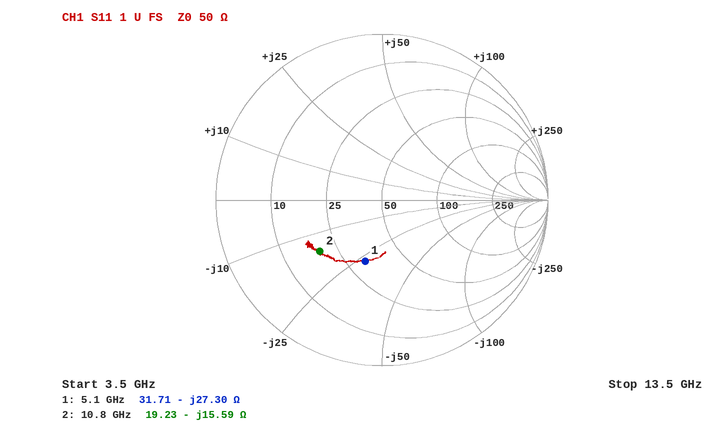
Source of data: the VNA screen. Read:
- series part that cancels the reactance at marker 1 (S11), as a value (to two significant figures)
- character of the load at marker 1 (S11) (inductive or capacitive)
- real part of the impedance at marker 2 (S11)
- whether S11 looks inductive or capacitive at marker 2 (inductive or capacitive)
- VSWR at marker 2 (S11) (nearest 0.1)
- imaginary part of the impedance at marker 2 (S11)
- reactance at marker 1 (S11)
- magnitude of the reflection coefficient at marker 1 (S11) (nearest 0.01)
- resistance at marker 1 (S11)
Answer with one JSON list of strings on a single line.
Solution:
["850 pH", "capacitive", "19.23 Ω", "capacitive", "2.9", "-15.59 Ω", "-27.30 Ω", "0.38", "31.71 Ω"]
